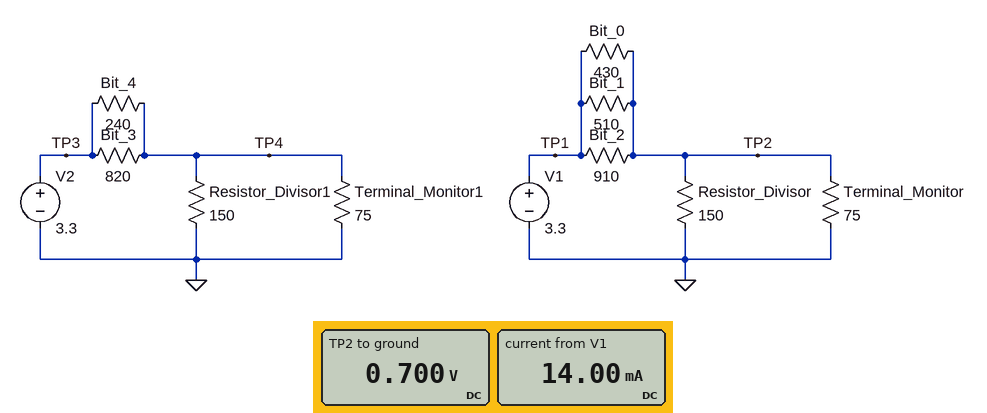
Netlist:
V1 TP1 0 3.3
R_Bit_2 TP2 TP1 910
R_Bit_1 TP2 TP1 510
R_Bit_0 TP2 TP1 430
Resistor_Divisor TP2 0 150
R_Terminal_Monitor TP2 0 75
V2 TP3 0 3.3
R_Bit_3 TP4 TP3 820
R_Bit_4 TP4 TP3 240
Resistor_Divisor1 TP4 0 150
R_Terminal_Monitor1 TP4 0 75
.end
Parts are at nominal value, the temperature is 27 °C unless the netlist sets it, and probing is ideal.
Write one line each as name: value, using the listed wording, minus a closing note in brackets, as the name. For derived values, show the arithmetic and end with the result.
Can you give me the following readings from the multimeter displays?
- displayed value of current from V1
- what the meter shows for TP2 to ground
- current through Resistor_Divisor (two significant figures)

displayed value of current from V1: 14.00 mA
what the meter shows for TP2 to ground: 0.700 V
current through Resistor_Divisor: (700 mV) / 150 Ω = 4.7 mA
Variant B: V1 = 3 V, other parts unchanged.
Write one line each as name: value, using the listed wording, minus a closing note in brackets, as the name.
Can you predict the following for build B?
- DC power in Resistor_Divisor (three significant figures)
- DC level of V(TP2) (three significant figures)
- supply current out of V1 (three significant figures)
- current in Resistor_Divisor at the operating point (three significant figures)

DC power in Resistor_Divisor: 2.70 mW
DC level of V(TP2): 636 mV
supply current out of V1: 12.7 mA
current in Resistor_Divisor at the operating point: 4.24 mA
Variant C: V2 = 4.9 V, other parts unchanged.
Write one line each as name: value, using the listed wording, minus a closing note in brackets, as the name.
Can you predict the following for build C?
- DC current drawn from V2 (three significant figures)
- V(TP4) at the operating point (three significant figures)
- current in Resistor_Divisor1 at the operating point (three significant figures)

DC current drawn from V2: 20.8 mA
V(TP4) at the operating point: 1.04 V
current in Resistor_Divisor1 at the operating point: 6.93 mA
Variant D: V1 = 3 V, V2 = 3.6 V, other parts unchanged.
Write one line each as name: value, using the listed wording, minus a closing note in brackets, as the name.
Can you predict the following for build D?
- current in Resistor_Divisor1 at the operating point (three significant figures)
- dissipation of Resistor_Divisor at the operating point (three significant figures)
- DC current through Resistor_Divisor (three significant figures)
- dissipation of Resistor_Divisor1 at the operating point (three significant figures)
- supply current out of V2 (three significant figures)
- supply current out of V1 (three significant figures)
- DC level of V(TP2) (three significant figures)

current in Resistor_Divisor1 at the operating point: 5.09 mA
dissipation of Resistor_Divisor at the operating point: 2.70 mW
DC current through Resistor_Divisor: 4.24 mA
dissipation of Resistor_Divisor1 at the operating point: 3.89 mW
supply current out of V2: 15.3 mA
supply current out of V1: 12.7 mA
DC level of V(TP2): 636 mV
